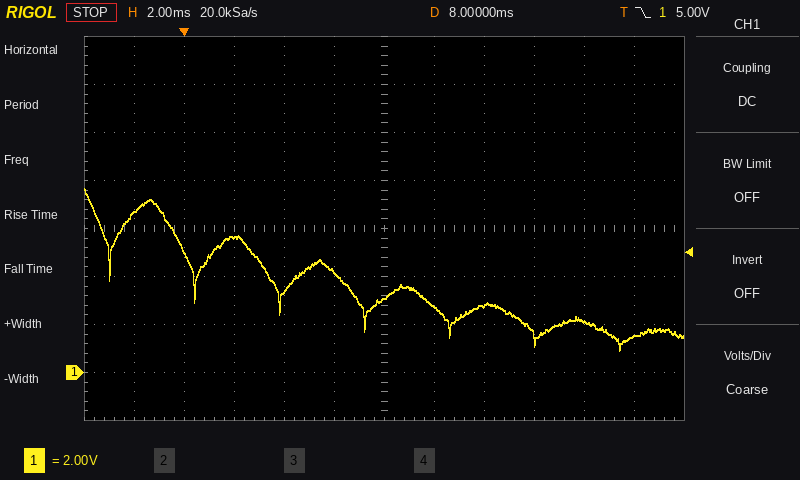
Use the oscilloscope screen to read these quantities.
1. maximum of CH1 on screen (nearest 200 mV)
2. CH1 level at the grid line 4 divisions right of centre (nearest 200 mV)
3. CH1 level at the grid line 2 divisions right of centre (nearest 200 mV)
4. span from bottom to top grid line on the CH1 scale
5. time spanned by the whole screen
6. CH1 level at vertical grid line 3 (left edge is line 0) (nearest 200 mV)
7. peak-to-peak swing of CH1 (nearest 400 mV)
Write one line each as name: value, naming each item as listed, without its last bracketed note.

maximum of CH1 on screen: 7.6 V
CH1 level at the grid line 4 divisions right of centre: 2.2 V
CH1 level at the grid line 2 divisions right of centre: 2.8 V
span from bottom to top grid line on the CH1 scale: 16 V
time spanned by the whole screen: 24 ms
CH1 level at vertical grid line 3 (left edge is line 0): 5.6 V
peak-to-peak swing of CH1: 6.8 V
